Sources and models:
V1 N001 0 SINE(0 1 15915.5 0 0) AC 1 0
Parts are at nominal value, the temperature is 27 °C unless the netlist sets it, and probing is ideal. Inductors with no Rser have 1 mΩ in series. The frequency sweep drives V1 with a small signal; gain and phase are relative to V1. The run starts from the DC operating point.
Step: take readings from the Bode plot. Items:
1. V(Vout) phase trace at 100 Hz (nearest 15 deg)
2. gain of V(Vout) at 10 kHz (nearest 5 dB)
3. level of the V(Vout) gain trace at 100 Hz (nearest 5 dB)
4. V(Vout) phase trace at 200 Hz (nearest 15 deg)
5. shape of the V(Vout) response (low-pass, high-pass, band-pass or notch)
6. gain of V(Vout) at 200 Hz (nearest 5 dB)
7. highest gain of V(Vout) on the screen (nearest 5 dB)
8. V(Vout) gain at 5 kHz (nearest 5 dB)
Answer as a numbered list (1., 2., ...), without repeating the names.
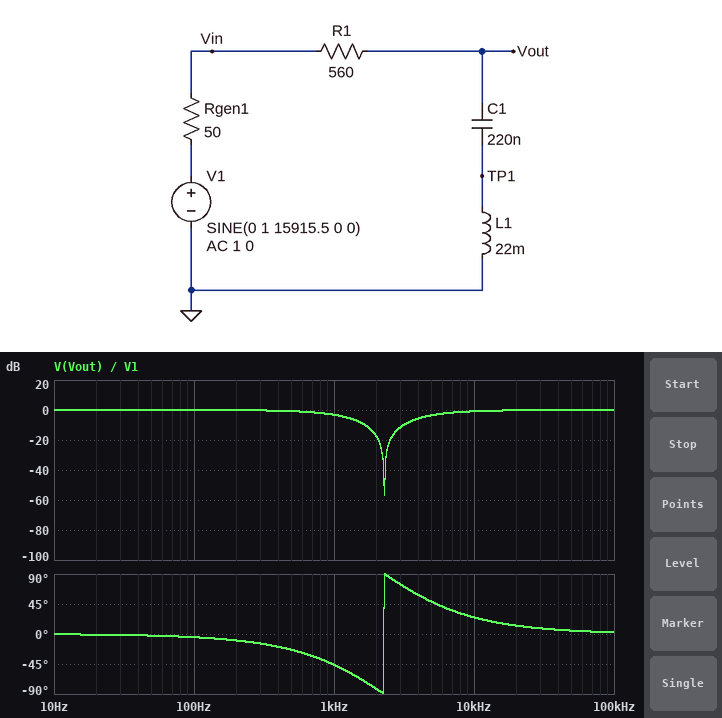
1. 0 deg
2. 0 dB
3. 0 dB
4. -15 deg
5. notch
6. 0 dB
7. 0 dB
8. -5 dB
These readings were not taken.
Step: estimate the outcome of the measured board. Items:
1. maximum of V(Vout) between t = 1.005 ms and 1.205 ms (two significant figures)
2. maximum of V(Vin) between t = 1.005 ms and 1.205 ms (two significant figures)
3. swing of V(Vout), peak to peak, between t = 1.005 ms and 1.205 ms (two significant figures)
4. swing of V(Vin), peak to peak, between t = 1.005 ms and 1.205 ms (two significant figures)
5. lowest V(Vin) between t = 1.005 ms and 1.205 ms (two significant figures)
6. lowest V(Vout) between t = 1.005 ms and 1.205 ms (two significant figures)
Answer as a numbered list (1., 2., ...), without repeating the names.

1. 960 mV
2. 990 mV
3. 1.9 V
4. 2.0 V
5. -990 mV
6. -960 mV
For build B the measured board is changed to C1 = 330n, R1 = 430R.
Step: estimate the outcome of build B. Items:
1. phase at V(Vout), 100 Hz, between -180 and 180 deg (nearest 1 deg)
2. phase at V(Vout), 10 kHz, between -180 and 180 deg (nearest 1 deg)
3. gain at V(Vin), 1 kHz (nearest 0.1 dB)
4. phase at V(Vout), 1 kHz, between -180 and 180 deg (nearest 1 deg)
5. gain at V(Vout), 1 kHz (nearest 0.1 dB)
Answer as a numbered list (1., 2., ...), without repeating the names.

1. -6 deg
2. 20 deg
3. -0.6 dB
4. -54 deg
5. -4.7 dB
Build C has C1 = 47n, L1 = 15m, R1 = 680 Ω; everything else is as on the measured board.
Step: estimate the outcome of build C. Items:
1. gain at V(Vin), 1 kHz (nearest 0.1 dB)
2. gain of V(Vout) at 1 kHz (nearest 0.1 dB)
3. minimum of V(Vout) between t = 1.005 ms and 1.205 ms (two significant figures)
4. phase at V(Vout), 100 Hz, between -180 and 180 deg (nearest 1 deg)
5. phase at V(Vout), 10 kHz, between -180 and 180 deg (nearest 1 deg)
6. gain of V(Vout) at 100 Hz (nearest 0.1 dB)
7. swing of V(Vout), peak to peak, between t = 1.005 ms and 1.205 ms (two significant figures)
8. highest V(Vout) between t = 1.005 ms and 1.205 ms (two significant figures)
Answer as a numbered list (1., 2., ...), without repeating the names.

1. 0 dB
2. -0.2 dB
3. -870 mV
4. -1 deg
5. 50 deg
6. 0 dB
7. 1.7 V
8. 870 mV
